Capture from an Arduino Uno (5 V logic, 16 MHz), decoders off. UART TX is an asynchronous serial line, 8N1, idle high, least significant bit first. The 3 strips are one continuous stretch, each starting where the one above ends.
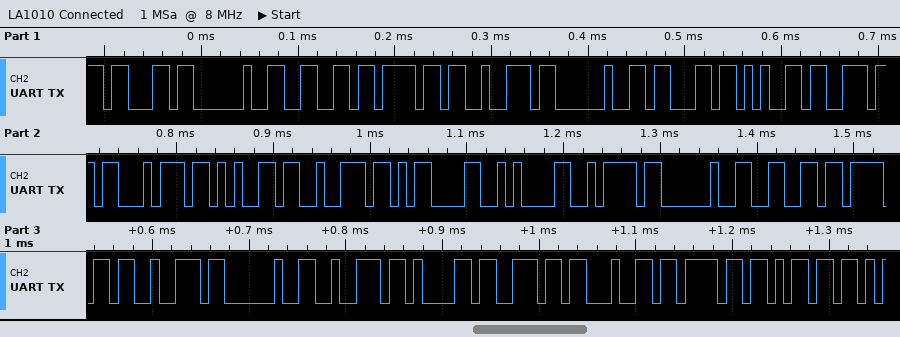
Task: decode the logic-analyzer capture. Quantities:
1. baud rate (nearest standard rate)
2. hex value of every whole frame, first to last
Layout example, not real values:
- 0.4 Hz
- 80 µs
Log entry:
- 115200 baud
- 63 20 66 6F 72 20 63 65 6E 74 65 72 0D 0A 7A 20 66 6F 72 20 72 61 6E 64 6F 6D
